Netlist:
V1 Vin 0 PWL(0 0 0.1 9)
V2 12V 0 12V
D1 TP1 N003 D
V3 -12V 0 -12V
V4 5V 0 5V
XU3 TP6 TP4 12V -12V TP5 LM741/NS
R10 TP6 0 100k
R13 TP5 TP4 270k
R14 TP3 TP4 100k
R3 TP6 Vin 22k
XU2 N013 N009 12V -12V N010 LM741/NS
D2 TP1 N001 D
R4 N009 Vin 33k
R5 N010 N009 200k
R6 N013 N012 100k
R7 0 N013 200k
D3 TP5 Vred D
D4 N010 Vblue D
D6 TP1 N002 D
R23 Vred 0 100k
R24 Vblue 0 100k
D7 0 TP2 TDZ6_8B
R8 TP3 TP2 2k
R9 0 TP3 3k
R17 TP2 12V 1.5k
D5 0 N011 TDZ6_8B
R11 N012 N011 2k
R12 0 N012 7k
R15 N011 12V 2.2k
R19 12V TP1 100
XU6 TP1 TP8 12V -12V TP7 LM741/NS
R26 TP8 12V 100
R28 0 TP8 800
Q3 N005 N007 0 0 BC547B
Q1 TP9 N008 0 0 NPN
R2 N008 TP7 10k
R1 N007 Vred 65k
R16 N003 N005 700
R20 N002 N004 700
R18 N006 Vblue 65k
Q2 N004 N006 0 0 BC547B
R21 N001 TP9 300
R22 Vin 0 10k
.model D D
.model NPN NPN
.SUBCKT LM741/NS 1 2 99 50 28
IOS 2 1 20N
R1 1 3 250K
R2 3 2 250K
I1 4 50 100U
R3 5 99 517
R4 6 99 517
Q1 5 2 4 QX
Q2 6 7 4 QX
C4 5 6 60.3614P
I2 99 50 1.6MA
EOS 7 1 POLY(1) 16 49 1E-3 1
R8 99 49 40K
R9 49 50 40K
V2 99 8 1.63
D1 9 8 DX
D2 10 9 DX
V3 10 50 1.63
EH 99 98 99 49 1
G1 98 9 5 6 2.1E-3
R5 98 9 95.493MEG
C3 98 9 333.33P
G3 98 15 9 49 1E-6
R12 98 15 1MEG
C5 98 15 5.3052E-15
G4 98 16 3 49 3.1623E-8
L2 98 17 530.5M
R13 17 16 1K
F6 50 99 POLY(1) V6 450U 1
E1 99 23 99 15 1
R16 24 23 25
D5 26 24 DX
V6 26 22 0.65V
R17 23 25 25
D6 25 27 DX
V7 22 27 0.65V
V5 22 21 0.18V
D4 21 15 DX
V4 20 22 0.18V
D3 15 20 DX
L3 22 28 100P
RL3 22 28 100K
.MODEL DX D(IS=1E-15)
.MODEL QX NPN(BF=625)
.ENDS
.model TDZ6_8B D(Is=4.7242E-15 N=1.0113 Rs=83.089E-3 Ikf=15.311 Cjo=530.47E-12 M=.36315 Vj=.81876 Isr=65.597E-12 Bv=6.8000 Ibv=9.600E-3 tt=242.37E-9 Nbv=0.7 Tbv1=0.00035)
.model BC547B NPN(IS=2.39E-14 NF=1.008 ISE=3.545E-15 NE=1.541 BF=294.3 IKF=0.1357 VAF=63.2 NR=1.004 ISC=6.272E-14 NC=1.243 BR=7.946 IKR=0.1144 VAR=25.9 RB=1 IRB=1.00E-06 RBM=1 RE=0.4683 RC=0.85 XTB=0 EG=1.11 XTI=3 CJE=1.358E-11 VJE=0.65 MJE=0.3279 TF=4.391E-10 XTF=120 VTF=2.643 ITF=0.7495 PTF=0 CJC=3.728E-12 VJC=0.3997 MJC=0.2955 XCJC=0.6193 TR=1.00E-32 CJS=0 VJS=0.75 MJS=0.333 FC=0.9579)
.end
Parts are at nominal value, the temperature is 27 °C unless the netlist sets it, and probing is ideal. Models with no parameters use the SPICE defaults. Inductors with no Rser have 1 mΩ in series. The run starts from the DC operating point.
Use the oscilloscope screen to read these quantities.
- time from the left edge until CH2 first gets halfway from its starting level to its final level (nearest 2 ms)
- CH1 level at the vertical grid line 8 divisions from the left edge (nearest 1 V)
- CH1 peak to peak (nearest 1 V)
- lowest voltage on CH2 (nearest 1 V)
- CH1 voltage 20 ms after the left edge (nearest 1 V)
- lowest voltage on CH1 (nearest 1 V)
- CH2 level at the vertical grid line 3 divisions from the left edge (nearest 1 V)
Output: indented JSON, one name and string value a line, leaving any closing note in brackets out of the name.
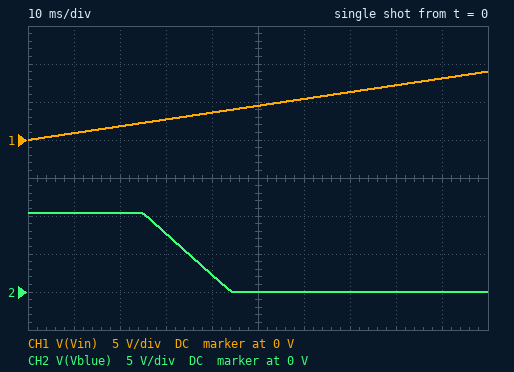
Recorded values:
{
  "time from the left edge until CH2 first gets halfway from its starting level to its final level": "34 ms",
  "CH1 level at the vertical grid line 8 divisions from the left edge": "7 V",
  "CH1 peak to peak": "9 V",
  "lowest voltage on CH2": "0 V",
  "CH1 voltage 20 ms after the left edge": "2 V",
  "lowest voltage on CH1": "0 V",
  "CH2 level at the vertical grid line 3 divisions from the left edge": "8 V"
}
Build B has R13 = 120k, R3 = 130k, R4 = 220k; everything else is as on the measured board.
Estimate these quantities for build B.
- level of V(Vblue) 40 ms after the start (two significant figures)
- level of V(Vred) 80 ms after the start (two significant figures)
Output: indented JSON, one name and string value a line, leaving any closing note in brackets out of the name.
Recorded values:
{
  "level of V(Vblue) 40 ms after the start": "2.8 V",
  "level of V(Vred) 80 ms after the start": "1.5 V"
}
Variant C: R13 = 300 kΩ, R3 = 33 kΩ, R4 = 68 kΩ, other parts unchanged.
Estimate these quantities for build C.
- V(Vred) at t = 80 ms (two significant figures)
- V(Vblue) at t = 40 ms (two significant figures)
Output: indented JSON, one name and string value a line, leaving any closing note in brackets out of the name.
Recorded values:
{
  "V(Vred) at t = 80 ms": "8.8 V",
  "V(Vblue) at t = 40 ms": "2.6 V"
}
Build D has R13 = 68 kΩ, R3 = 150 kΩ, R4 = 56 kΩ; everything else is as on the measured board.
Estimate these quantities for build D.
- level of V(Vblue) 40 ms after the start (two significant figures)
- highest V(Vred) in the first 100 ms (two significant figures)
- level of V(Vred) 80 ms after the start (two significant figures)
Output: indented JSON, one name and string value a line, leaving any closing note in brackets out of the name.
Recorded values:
{
  "level of V(Vblue) 40 ms after the start": "2.5 V",
  "highest V(Vred) in the first 100 ms": "2.7 V",
  "level of V(Vred) 80 ms after the start": "1.5 V"
}
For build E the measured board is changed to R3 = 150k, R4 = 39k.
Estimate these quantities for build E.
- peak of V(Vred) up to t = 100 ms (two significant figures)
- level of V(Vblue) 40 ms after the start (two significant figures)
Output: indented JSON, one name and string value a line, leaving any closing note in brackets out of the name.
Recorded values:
{
  "peak of V(Vred) up to t = 100 ms": "1.8 V",
  "level of V(Vblue) 40 ms after the start": "2.4 V"
}
